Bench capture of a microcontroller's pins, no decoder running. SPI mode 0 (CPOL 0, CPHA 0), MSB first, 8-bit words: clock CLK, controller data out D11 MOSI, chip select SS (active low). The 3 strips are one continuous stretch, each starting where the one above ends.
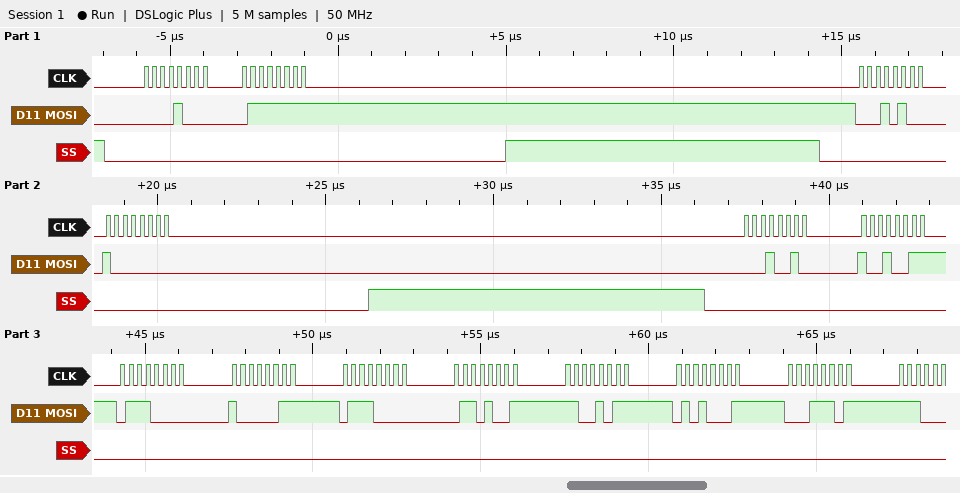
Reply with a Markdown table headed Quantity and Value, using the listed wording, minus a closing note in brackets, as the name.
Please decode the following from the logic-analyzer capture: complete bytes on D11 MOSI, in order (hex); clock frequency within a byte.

| Quantity | Value |
|---|---|
| complete bytes on D11 MOSI, in order | 0x08 0x7F 0x14 0x80 0x12 0x93 0x70 0x83 0x70 0x69 0xCB 0x51 0x1D |
| clock frequency within a byte | 4 MHz |
